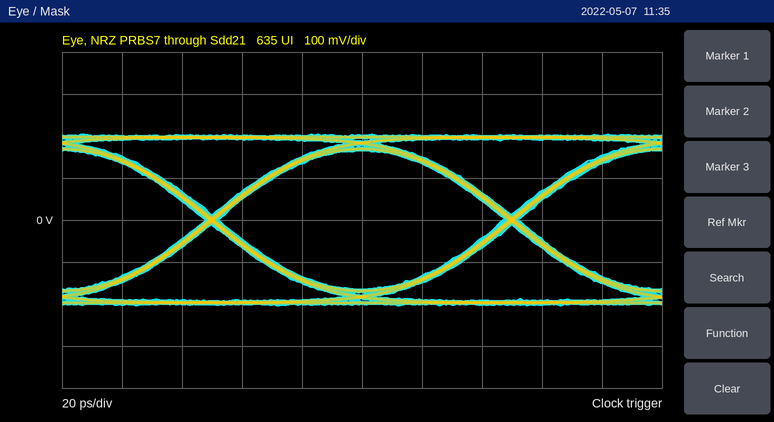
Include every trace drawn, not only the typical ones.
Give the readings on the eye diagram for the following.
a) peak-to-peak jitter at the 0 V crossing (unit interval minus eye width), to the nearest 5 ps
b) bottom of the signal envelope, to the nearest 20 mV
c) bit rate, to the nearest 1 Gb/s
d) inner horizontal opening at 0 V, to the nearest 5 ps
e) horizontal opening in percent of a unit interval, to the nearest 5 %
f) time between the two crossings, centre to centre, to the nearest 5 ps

5 ps
-200 mV
10 Gb/s
95 ps
95 %
100 ps
